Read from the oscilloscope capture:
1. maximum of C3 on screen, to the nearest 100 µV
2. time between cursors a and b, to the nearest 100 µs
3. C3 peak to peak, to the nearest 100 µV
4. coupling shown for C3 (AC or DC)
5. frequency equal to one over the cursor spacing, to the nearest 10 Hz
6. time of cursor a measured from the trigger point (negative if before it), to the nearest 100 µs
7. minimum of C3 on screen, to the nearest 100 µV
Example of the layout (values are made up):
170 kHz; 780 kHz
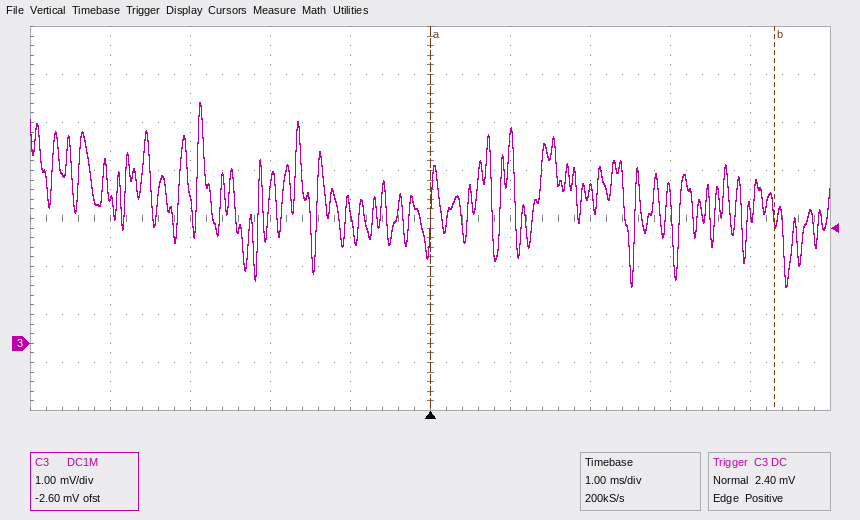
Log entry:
5.0 mV; 4.3 ms; 3.8 mV; DC; 230 Hz; 0.0 ms; 1.2 mV
